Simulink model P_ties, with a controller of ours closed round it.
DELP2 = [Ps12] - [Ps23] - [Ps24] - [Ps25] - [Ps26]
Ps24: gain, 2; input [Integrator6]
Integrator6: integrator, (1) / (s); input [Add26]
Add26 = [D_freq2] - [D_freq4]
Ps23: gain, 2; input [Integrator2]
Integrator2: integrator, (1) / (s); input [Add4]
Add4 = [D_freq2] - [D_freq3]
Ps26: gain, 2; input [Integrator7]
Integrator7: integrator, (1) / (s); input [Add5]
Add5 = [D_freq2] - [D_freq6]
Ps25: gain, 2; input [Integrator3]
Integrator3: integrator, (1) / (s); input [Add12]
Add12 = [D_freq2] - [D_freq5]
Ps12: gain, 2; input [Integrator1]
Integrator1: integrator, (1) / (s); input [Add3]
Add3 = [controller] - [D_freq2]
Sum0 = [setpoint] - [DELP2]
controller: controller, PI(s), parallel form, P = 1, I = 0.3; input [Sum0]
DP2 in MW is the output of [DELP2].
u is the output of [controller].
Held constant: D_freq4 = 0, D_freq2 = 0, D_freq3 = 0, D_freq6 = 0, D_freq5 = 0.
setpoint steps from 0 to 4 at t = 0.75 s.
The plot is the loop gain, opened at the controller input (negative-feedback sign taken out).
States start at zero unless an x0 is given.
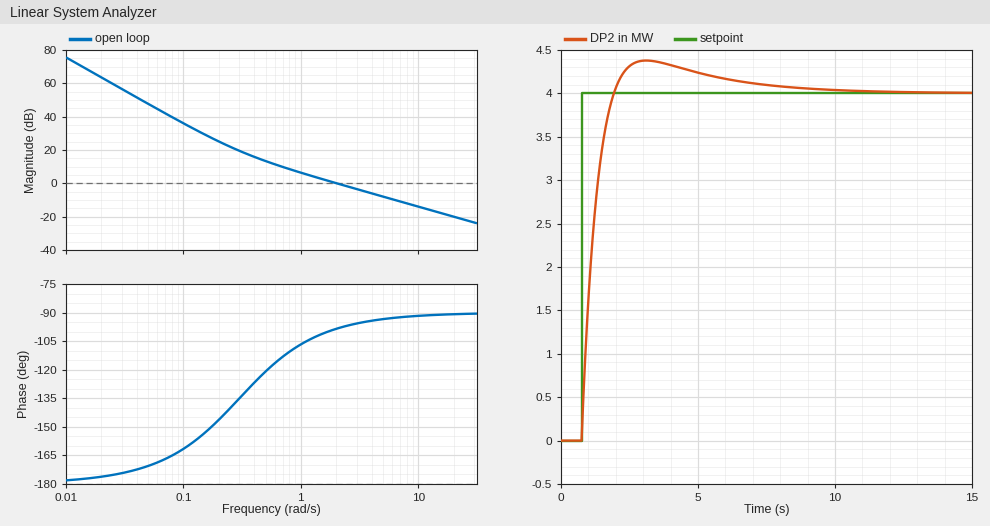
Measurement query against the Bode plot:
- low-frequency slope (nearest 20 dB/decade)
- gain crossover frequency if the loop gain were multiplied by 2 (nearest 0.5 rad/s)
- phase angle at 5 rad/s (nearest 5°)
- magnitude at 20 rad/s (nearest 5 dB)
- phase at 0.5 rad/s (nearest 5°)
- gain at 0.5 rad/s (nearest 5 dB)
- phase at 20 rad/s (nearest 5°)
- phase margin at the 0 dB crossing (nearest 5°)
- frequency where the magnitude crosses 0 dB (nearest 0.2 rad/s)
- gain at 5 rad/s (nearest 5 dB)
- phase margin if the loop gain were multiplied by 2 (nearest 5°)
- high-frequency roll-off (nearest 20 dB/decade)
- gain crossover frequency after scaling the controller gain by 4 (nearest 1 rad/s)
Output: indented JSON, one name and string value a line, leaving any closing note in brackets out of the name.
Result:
{
  "low-frequency slope": "-40 dB/decade",
  "gain crossover frequency if the loop gain were multiplied by 2": "4.0 rad/s",
  "phase angle at 5 rad/s": "-95°",
  "magnitude at 20 rad/s": "-20 dB",
  "phase at 0.5 rad/s": "-120°",
  "gain at 0.5 rad/s": "15 dB",
  "phase at 20 rad/s": "-90°",
  "phase margin at the 0 dB crossing": "80°",
  "frequency where the magnitude crosses 0 dB": "2.0 rad/s",
  "gain at 5 rad/s": "-10 dB",
  "phase margin if the loop gain were multiplied by 2": "85°",
  "high-frequency roll-off": "-20 dB/decade",
  "gain crossover frequency after scaling the controller gain by 4": "8 rad/s"
}
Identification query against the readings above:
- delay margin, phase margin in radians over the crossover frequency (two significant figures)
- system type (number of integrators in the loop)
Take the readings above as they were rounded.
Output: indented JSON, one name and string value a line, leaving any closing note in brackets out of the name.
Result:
{
  "delay margin, phase margin in radians over the crossover frequency": "0.70 s",
  "system type": "2"
}
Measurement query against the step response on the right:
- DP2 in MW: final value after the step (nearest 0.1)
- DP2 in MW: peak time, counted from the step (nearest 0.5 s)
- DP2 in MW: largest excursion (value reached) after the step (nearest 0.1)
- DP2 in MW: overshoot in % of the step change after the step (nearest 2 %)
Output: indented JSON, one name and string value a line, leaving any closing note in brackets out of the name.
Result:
{
  "DP2 in MW: final value after the step": "4.0",
  "DP2 in MW: peak time, counted from the step": "2.5 s",
  "DP2 in MW: largest excursion (value reached) after the step": "4.4",
  "DP2 in MW: overshoot in % of the step change after the step": "10 %"
}
